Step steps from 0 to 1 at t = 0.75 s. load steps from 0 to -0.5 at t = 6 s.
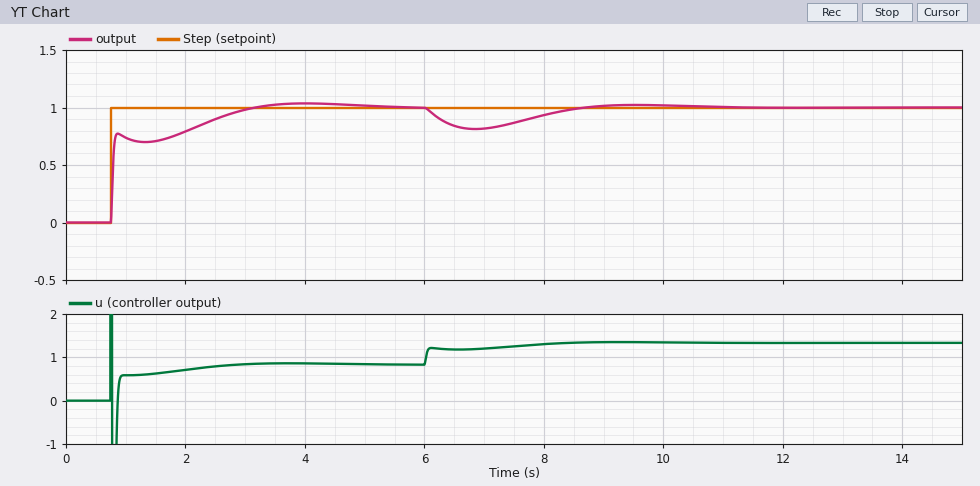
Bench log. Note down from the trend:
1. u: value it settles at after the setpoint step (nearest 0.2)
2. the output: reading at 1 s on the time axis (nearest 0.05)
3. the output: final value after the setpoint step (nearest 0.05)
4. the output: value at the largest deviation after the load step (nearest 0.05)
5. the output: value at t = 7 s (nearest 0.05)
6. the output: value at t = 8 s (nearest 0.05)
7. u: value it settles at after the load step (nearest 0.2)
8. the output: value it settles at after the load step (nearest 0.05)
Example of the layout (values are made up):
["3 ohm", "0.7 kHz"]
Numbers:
["0.8", "0.75", "1.00", "0.80", "0.80", "0.95", "1.4", "1.00"]
